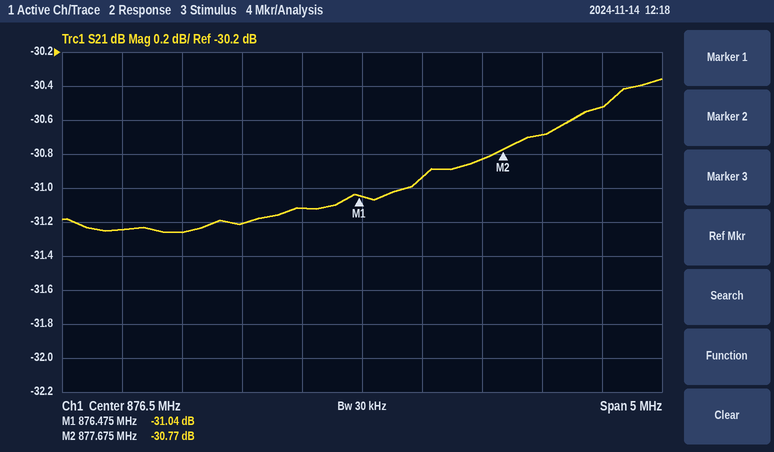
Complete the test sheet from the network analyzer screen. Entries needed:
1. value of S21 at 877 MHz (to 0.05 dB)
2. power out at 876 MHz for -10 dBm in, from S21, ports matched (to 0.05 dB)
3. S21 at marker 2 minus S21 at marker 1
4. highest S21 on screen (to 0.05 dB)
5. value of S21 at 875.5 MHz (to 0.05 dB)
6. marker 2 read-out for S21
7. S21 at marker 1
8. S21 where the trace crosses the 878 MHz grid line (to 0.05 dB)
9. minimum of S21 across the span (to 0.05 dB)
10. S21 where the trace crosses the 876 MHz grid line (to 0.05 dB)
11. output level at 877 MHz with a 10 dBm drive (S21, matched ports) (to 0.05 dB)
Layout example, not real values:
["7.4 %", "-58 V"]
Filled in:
["-30.95 dB", "-41.10 dBm", "0.27 dB", "-30.35 dB", "-31.20 dB", "-30.77 dB", "-31.04 dB", "-30.70 dB", "-31.25 dB", "-31.10 dB", "-20.95 dBm"]
